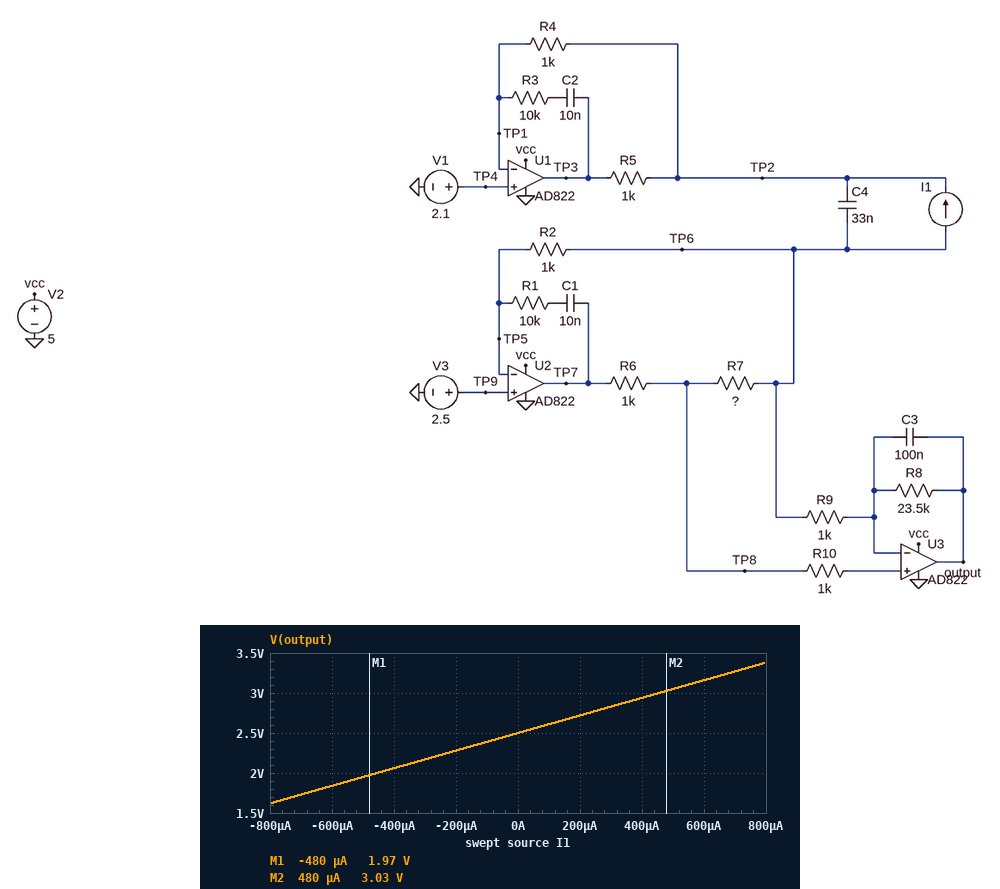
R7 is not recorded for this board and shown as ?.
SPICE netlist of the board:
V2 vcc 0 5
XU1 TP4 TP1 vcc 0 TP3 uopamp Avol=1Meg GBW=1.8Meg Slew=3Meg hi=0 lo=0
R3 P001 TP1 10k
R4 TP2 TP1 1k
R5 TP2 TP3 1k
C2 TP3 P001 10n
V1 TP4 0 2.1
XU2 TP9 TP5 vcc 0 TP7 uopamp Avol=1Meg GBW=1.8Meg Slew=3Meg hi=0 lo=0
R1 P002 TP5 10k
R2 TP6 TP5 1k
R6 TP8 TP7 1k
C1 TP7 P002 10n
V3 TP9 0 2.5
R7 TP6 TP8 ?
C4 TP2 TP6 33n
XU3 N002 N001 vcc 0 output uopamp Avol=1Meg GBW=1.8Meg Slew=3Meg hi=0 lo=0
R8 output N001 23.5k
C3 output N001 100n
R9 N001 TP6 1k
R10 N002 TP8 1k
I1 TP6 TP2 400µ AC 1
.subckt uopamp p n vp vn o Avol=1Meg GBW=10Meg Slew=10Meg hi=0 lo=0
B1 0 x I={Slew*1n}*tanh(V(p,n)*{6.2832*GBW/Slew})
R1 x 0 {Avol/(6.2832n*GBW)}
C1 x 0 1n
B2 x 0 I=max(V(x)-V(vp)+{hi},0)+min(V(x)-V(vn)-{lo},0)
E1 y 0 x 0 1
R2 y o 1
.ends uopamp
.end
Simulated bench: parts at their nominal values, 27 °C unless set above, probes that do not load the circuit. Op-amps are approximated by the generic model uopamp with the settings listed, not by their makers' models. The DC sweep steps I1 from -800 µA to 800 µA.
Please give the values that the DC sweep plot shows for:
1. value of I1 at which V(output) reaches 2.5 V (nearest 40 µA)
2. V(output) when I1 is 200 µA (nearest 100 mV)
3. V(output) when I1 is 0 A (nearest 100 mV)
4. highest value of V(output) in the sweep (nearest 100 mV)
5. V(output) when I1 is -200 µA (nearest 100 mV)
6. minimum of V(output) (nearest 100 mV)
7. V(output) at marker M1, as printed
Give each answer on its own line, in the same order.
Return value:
0 A
2.7 V
2.5 V
3.4 V
2.3 V
1.6 V
1.97 V
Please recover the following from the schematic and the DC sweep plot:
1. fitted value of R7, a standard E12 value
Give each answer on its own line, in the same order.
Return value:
47 Ω
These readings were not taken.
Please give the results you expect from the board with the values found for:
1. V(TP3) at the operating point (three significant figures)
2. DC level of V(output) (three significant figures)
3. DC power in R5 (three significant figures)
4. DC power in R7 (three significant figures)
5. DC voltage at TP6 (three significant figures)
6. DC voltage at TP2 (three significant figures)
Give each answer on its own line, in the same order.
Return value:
1.70 V
2.94 V
160 µW
6.86 µW
2.50 V
2.10 V
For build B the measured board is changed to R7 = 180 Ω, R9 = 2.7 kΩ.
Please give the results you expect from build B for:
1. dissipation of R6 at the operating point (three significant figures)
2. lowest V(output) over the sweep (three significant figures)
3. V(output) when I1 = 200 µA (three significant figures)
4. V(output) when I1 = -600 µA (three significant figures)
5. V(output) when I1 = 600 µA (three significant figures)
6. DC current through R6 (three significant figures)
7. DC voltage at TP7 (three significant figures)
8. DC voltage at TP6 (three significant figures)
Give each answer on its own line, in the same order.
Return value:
141 µW
1.19 V
2.83 V
1.52 V
3.48 V
375 µA
2.94 V
2.50 V
